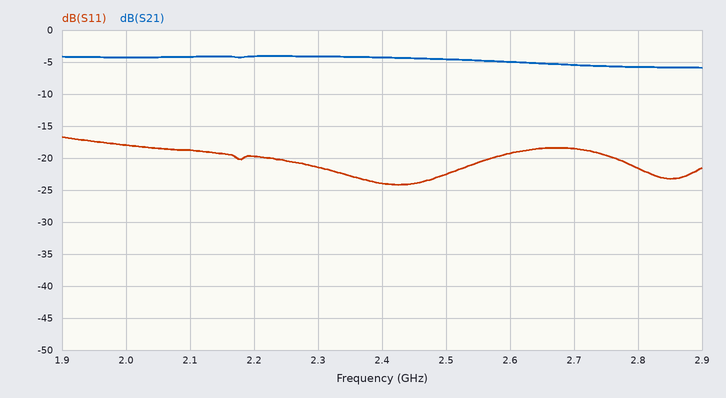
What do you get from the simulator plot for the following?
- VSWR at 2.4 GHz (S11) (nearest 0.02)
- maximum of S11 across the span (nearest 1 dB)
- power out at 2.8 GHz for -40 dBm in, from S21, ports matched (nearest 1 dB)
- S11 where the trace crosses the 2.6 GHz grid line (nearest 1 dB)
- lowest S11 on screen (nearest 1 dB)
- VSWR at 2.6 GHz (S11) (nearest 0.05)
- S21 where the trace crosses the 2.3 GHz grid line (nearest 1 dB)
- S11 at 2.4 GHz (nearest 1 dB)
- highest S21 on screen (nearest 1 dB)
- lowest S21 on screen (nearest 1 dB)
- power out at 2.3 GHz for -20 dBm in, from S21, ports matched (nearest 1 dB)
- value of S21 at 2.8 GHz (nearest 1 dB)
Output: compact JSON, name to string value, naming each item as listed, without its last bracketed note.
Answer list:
{"VSWR at 2.4 GHz (S11)": "1.14", "maximum of S11 across the span": "-17 dB", "power out at 2.8 GHz for -40 dBm in, from S21, ports matched": "-46 dBm", "S11 where the trace crosses the 2.6 GHz grid line": "-19 dB", "lowest S11 on screen": "-24 dB", "VSWR at 2.6 GHz (S11)": "1.25", "S21 where the trace crosses the 2.3 GHz grid line": "-4 dB", "S11 at 2.4 GHz": "-24 dB", "highest S21 on screen": "-4 dB", "lowest S21 on screen": "-6 dB", "power out at 2.3 GHz for -20 dBm in, from S21, ports matched": "-24 dBm", "value of S21 at 2.8 GHz": "-6 dB"}
